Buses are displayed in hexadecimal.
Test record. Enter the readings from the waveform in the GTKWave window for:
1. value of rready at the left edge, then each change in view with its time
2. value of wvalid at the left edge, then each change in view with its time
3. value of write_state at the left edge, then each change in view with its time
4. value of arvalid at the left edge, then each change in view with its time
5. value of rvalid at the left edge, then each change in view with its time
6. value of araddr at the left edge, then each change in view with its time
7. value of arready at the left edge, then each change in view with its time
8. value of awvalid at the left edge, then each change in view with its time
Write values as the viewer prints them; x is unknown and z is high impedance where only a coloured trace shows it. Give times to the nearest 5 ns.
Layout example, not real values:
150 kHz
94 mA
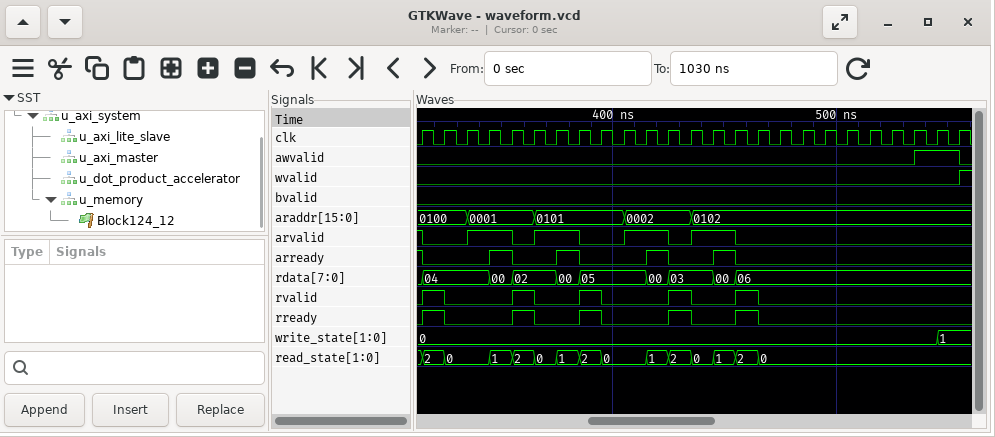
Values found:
0, 1 at 315 ns, 0 at 325 ns, 1 at 355 ns, 0 at 365 ns, 1 at 385 ns, 0 at 395 ns, 1 at 425 ns, 0 at 435 ns, 1 at 455 ns, 0 at 465 ns
0, 1 at 555 ns
0, 1 at 545 ns
1, 0 at 315 ns, 1 at 335 ns, 0 at 355 ns, 1 at 365 ns, 0 at 385 ns, 1 at 405 ns, 0 at 425 ns, 1 at 435 ns, 0 at 455 ns
0, 1 at 315 ns, 0 at 325 ns, 1 at 355 ns, 0 at 365 ns, 1 at 385 ns, 0 at 395 ns, 1 at 425 ns, 0 at 435 ns, 1 at 455 ns, 0 at 465 ns
0100, 0001 at 335 ns, 0101 at 365 ns, 0002 at 405 ns, 0102 at 435 ns
1, 0 at 315 ns, 1 at 345 ns, 0 at 355 ns, 1 at 375 ns, 0 at 385 ns, 1 at 415 ns, 0 at 425 ns, 1 at 445 ns, 0 at 455 ns
0, 1 at 535 ns, 0 at 555 ns
